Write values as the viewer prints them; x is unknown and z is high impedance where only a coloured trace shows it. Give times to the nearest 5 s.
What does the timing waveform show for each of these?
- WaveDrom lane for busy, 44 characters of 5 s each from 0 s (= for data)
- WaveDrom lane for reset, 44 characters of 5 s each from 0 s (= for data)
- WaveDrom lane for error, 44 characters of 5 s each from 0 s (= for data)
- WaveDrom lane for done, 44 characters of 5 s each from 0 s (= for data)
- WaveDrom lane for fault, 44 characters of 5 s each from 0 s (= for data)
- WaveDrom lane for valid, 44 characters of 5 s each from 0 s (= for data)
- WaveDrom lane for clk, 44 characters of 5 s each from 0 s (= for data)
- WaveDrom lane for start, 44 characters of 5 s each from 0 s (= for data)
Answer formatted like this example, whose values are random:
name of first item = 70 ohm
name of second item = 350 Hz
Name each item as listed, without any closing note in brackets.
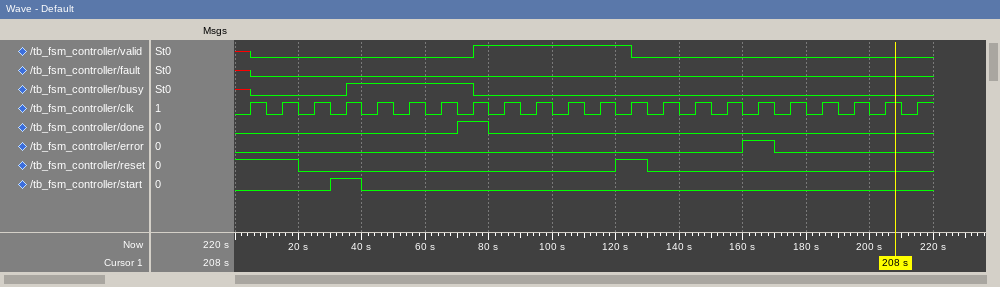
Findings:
WaveDrom lane for busy, 44 characters of 5 s each from 0 s = {name: 'busy', wave: 'x0.....1.......0............................'}
WaveDrom lane for reset, 44 characters of 5 s each from 0 s = {name: 'reset', wave: '1...0...................1.0.................'}
WaveDrom lane for error, 44 characters of 5 s each from 0 s = {name: 'error', wave: '0...............................1.0.........'}
WaveDrom lane for done, 44 characters of 5 s each from 0 s = {name: 'done', wave: '0.............1.0...........................'}
WaveDrom lane for fault, 44 characters of 5 s each from 0 s = {name: 'fault', wave: 'x0..........................................'}
WaveDrom lane for valid, 44 characters of 5 s each from 0 s = {name: 'valid', wave: 'x0.............1.........0..................'}
WaveDrom lane for clk, 44 characters of 5 s each from 0 s = {name: 'clk', wave: '01010101010101010101010101010101010101010101'}
WaveDrom lane for start, 44 characters of 5 s each from 0 s = {name: 'start', wave: '0.....1.0...................................'}
